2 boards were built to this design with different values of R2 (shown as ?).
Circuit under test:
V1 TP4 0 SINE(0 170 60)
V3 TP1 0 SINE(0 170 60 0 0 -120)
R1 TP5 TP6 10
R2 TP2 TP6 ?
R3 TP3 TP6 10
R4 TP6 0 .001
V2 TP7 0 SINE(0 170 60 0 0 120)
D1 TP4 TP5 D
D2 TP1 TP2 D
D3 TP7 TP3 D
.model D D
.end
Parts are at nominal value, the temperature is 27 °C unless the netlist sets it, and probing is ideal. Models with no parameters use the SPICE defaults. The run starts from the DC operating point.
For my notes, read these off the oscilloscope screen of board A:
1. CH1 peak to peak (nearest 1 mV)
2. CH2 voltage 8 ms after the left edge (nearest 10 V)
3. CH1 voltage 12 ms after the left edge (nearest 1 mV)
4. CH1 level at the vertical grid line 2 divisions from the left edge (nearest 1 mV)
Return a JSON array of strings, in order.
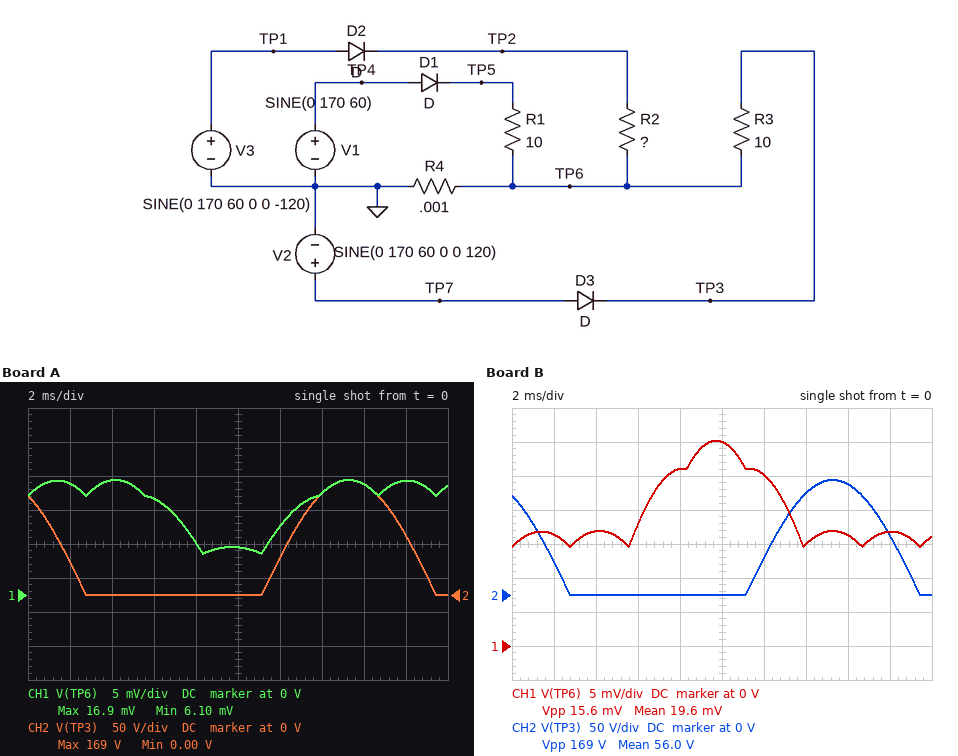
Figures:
["11 mV", "0 V", "10 mV", "17 mV"]
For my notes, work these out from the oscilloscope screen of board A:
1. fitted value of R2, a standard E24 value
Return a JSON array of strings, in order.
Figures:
["24 Ω"]
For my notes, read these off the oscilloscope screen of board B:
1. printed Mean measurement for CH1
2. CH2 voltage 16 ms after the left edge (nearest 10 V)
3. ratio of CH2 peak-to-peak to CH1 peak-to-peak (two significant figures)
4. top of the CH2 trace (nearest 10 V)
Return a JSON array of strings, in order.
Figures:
["19.6 mV", "160 V", "11000", "170 V"]
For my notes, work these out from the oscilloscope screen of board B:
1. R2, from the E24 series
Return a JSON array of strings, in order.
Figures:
["5.6 Ω"]
